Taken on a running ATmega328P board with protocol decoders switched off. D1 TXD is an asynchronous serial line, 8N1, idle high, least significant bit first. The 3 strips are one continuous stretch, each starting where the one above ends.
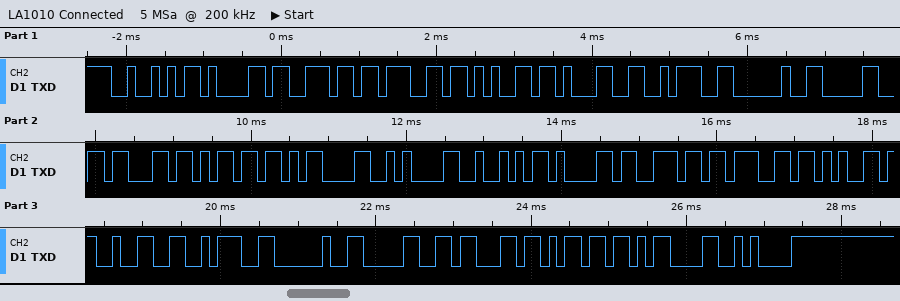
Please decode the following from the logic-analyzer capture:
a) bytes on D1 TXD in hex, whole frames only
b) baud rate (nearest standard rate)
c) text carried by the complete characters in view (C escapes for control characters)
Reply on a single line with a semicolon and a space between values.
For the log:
52 61 6E 67 65 31 3A 20 30 63 6D 0D 0A 52 61 6E 67 65 32 3A 20 30 63 6D 0D 0A; 9600 baud; "Range1: 0cm\r\nRange2: 0cm\r\n"
